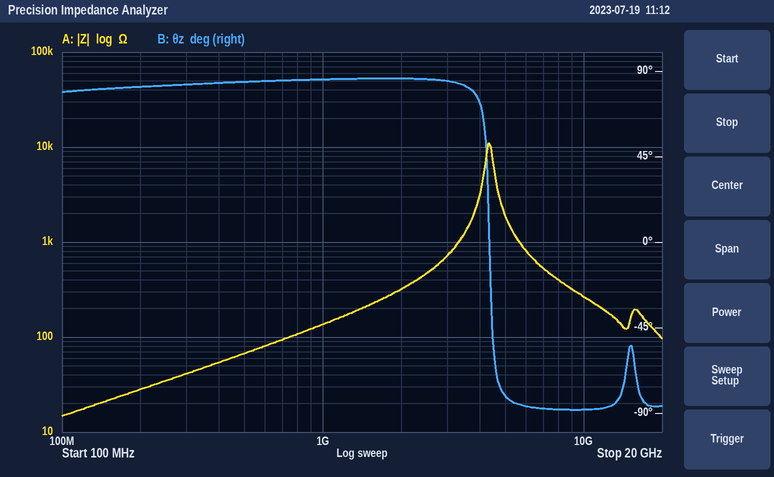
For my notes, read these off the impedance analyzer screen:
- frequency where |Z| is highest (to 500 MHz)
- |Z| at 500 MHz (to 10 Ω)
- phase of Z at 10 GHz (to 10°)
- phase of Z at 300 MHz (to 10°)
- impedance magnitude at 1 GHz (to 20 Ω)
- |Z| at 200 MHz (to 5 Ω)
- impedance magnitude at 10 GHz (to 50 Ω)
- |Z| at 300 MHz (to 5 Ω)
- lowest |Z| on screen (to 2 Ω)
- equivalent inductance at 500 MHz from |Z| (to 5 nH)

4.5 GHz
70 Ω
-90°
80°
140 Ω
30 Ω
250 Ω
40 Ω
14 Ω
20 nH
